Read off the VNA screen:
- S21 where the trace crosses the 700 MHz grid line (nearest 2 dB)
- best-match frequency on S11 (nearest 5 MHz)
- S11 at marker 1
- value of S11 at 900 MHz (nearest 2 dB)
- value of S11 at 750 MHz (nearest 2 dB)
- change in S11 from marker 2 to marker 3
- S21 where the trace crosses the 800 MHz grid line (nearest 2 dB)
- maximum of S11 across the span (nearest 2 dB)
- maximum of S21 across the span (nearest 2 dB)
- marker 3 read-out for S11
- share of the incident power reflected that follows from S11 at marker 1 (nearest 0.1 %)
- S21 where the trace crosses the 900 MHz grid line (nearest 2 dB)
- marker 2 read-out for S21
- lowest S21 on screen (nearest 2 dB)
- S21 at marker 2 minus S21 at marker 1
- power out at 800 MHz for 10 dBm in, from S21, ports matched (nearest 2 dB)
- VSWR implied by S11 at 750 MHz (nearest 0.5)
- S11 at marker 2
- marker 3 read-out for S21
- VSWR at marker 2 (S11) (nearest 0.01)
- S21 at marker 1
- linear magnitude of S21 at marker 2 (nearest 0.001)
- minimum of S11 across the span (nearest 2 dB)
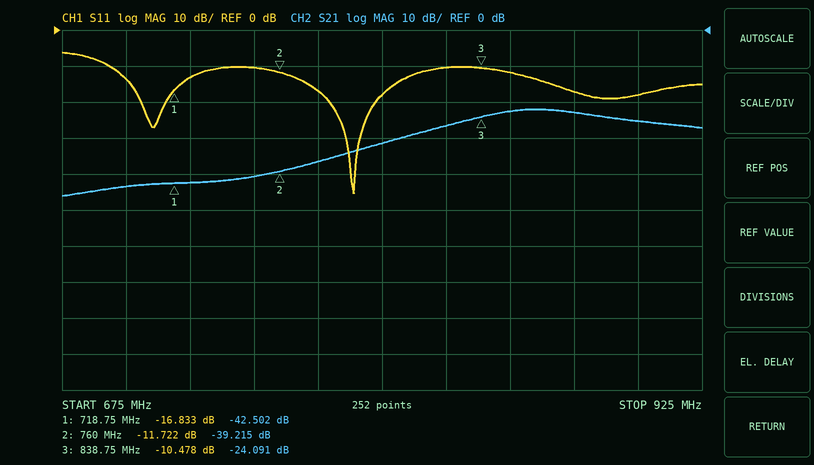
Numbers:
-44 dB
790 MHz
-16.833 dB
-18 dB
-10 dB
1.244 dB
-32 dB
-6 dB
-22 dB
-10.478 dB
2.1 %
-26 dB
-39.215 dB
-46 dB
3.287 dB
-22 dBm
2.0
-11.722 dB
-24.091 dB
1.70
-42.502 dB
0.011
-46 dB
